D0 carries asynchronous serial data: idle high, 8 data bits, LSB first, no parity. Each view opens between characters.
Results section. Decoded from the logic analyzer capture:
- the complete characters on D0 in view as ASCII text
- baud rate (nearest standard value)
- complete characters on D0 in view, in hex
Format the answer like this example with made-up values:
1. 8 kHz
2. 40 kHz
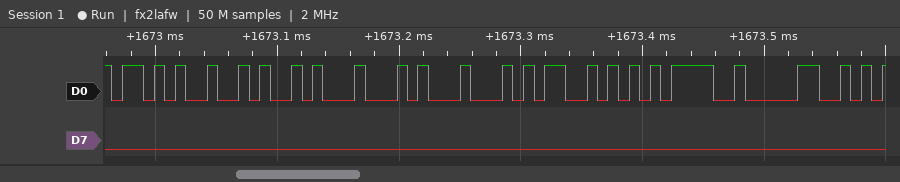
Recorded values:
1. "+JDDS=0"
2. 115200 baud
3. 2B, 4A, 44, 44, 53, 3D, 30
